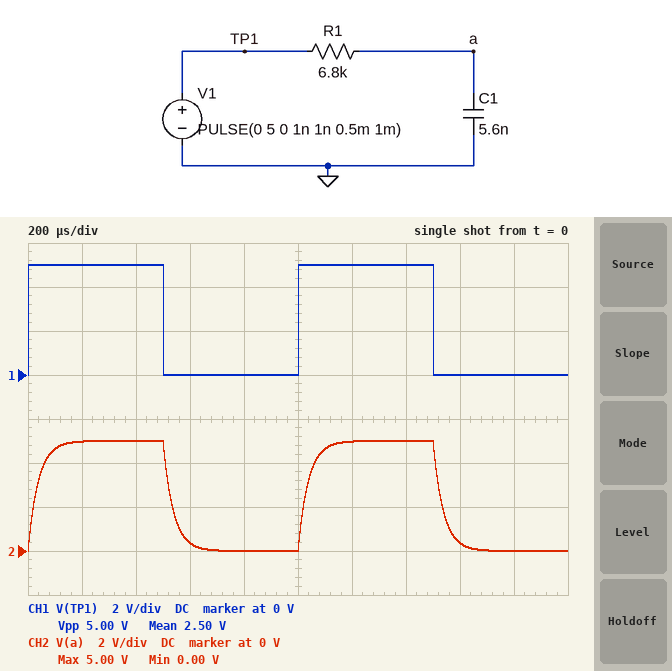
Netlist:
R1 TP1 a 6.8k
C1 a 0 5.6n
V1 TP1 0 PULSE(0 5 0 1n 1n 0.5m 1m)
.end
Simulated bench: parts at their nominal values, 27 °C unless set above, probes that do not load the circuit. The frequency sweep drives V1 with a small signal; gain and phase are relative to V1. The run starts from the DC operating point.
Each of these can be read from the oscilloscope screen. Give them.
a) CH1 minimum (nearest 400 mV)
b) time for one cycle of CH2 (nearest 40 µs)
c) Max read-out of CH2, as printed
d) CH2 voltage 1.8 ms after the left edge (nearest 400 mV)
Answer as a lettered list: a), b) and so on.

a) 0 V
b) 1.00 ms
c) 5.00 V
d) 0 V
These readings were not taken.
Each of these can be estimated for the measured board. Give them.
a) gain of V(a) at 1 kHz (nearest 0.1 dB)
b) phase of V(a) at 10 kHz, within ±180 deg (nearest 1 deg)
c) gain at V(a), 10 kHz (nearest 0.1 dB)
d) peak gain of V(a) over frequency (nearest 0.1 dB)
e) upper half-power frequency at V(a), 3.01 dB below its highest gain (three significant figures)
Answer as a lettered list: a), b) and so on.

a) -0.2 dB
b) -67 deg
c) -8.3 dB
d) 0 dB
e) 4.18 kHz
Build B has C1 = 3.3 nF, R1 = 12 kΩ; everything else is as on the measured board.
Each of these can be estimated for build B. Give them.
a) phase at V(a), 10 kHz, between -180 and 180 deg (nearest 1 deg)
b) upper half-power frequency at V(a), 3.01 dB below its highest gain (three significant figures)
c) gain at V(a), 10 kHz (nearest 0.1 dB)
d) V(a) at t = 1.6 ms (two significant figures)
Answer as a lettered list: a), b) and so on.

a) -68 deg
b) 4.02 kHz
c) -8.6 dB
d) 400 mV
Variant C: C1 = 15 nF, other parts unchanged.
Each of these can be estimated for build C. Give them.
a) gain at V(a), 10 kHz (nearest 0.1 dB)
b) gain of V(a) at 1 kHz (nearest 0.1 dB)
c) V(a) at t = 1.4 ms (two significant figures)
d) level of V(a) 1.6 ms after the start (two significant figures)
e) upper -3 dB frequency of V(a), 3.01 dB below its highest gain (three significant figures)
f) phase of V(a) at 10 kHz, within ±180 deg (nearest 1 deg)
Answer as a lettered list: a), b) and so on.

a) -16.2 dB
b) -1.5 dB
c) 4.9 V
d) 1.9 V
e) 1.56 kHz
f) -81 deg
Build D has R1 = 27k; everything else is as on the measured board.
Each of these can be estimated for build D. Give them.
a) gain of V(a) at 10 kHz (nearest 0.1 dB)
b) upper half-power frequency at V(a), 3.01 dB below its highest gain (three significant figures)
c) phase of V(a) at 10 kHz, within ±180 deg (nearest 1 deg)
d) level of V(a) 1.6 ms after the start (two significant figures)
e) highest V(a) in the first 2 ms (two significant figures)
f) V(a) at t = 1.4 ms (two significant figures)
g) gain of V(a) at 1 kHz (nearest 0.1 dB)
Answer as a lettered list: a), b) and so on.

a) -19.6 dB
b) 1.05 kHz
c) -84 deg
d) 2.5 V
e) 4.8 V
f) 4.7 V
g) -2.8 dB
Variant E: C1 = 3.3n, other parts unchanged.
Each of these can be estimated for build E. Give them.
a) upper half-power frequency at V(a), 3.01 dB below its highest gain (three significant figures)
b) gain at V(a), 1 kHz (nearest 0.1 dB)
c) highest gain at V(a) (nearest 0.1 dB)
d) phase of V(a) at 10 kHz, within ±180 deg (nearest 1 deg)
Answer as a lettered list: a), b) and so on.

a) 7.09 kHz
b) -0.1 dB
c) 0 dB
d) -55 deg
